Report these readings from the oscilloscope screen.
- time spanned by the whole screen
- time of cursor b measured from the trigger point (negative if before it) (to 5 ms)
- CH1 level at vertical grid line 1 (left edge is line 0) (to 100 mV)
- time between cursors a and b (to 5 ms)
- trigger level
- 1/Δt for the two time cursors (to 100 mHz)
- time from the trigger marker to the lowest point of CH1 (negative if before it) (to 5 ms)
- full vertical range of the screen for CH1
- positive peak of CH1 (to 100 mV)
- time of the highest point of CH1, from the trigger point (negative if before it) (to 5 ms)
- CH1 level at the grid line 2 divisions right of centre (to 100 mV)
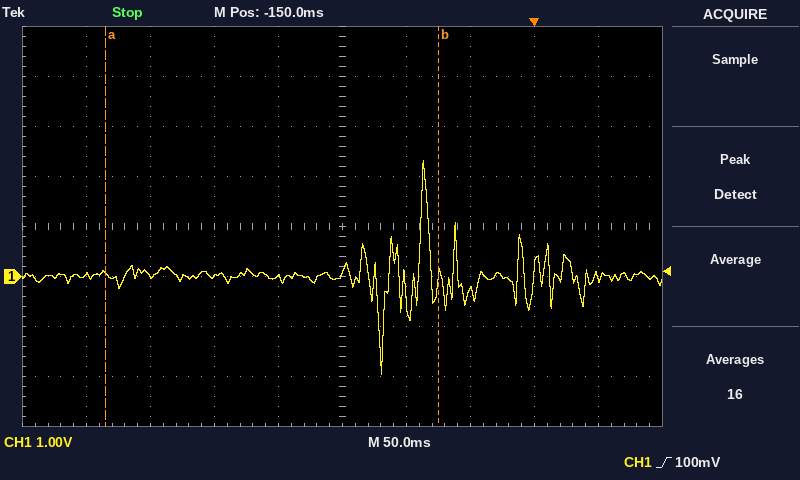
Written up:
500 ms
-75 ms
0.0 V
260 ms
100 mV
3.8 Hz
-120 ms
8 V
2.3 V
-85 ms
-300 mV
